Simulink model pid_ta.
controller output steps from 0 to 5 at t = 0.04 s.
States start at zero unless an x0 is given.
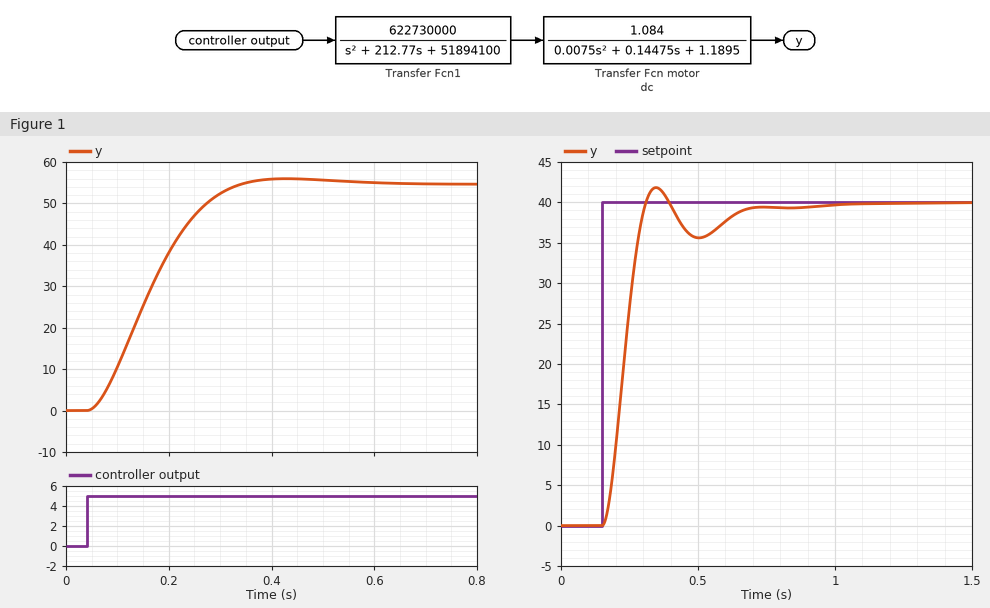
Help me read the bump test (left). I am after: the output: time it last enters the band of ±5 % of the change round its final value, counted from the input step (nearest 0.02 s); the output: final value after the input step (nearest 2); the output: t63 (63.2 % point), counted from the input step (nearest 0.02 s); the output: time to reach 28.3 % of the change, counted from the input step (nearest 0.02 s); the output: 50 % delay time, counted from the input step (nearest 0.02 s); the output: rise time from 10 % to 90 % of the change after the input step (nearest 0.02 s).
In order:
0.26 s
54
0.14 s
0.08 s
0.12 s
0.18 s
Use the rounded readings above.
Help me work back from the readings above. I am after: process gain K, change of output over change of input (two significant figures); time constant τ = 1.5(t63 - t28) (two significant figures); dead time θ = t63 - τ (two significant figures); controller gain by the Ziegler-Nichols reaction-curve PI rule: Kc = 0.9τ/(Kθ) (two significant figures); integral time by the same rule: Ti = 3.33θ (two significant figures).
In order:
11
0.090 s
0.050 s
0.15
0.17 s
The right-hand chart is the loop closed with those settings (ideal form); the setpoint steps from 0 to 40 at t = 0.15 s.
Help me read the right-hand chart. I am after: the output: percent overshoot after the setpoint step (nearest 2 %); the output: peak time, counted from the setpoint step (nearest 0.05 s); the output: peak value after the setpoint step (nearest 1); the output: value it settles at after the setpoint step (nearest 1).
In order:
4 %
0.20 s
42
40
